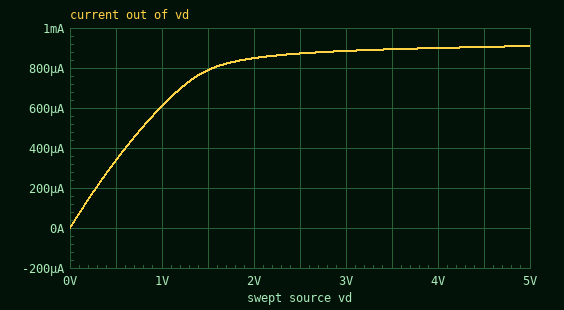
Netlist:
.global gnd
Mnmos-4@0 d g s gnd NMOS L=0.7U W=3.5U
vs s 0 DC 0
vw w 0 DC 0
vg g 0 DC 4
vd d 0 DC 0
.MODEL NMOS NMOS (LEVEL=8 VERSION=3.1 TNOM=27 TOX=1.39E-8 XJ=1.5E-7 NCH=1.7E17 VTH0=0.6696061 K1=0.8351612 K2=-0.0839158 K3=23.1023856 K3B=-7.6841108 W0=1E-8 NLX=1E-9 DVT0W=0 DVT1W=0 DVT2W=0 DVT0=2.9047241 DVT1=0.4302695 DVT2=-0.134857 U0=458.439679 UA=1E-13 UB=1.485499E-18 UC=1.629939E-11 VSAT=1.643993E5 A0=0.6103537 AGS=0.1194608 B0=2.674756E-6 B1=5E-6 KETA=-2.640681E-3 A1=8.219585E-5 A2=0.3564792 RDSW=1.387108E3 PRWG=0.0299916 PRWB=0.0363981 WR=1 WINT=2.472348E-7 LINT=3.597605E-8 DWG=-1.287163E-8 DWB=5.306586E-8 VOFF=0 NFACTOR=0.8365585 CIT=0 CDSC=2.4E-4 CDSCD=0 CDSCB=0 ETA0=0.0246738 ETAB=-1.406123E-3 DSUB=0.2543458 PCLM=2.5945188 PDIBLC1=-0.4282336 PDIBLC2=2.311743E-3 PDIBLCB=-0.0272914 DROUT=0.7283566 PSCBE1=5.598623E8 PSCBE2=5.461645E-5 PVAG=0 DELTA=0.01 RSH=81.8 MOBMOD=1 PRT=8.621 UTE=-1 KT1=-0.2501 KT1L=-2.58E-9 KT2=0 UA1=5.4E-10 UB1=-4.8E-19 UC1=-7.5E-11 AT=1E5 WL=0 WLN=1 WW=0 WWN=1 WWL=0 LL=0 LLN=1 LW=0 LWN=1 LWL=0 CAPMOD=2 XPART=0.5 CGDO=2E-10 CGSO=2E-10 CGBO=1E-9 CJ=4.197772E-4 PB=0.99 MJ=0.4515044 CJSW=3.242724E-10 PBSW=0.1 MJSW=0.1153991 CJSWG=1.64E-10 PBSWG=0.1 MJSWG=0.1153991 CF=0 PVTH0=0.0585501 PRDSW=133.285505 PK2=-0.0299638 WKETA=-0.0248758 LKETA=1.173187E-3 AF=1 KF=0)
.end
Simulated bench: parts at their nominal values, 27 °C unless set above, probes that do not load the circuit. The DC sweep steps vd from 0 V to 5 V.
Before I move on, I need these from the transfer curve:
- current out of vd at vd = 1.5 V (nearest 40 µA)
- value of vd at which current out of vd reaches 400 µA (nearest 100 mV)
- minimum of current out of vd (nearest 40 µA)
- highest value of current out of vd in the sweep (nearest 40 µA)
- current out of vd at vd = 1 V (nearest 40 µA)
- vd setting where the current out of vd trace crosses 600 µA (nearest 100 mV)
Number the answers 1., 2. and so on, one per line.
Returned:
1. 800 µA
2. 600 mV
3. 0 A
4. 920 µA
5. 600 µA
6. 1.0 V
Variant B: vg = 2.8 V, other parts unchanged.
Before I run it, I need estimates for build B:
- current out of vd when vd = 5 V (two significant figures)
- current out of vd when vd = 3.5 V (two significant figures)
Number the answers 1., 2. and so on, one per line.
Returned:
1. 520 µA
2. 510 µA
